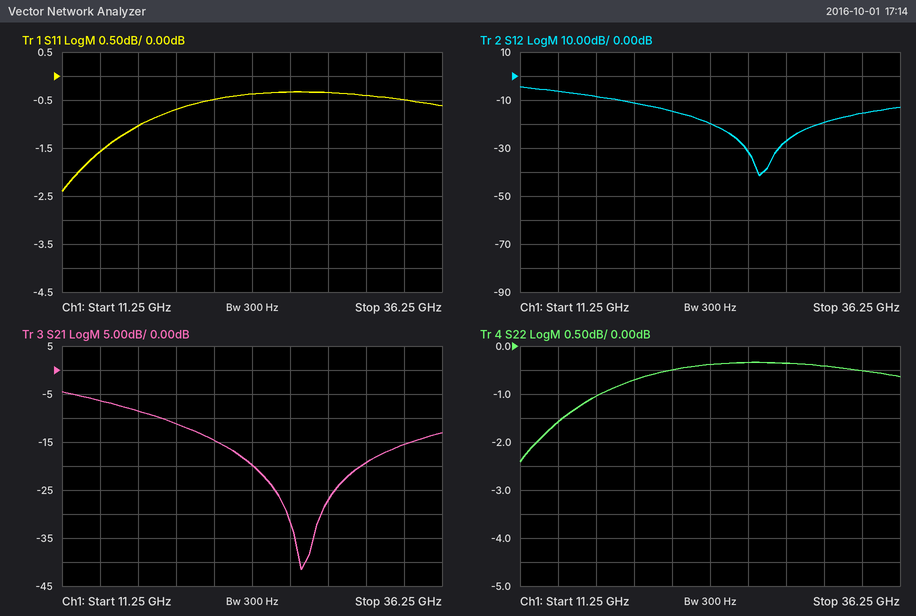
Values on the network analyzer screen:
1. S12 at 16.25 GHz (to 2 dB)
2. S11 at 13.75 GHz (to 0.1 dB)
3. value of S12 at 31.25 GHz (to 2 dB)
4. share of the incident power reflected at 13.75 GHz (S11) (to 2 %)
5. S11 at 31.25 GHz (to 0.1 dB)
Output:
-8 dB
-1.6 dB
-20 dB
70 %
-0.4 dB
